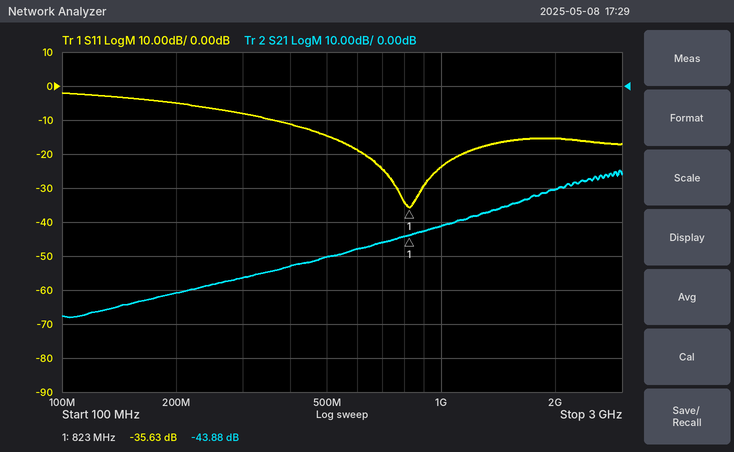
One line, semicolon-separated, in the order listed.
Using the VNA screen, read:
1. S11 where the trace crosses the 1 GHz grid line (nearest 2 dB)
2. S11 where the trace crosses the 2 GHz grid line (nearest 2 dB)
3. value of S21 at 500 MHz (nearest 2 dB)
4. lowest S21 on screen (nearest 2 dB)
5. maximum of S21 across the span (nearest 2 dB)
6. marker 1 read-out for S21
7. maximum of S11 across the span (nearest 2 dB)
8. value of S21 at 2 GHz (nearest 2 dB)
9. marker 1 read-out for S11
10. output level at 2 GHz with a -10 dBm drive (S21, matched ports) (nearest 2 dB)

-24 dB; -16 dB; -50 dB; -68 dB; -24 dB; -43.88 dB; -2 dB; -30 dB; -35.63 dB; -40 dBm
